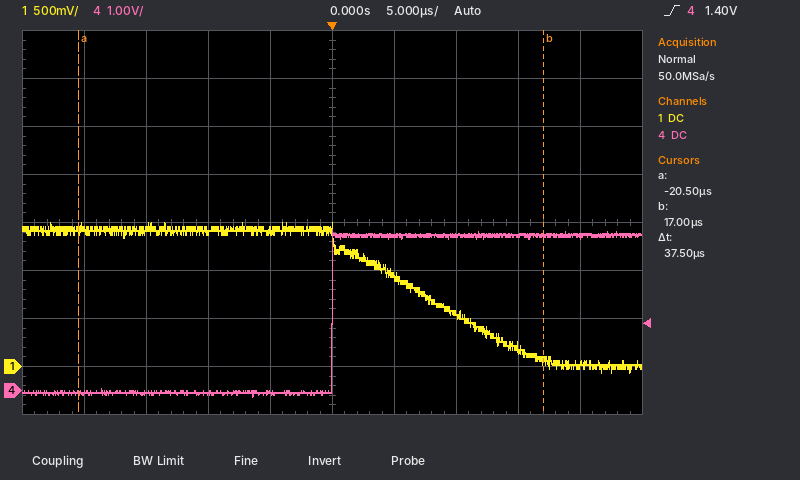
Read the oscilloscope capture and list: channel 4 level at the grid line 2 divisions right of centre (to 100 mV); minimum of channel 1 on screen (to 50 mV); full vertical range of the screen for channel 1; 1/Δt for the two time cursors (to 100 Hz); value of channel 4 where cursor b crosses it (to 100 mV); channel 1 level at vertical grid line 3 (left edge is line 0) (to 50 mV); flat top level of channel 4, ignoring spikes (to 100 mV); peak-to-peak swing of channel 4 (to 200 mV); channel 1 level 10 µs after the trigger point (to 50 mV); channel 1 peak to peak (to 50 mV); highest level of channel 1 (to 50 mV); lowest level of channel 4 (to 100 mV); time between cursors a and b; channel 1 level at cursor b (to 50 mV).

3.2 V
-50 mV
4 V
26.7 kHz
3.2 V
1.40 V
3.2 V
3.4 V
550 mV
1.55 V
1.50 V
-100 mV
37.5 µs
50 mV
